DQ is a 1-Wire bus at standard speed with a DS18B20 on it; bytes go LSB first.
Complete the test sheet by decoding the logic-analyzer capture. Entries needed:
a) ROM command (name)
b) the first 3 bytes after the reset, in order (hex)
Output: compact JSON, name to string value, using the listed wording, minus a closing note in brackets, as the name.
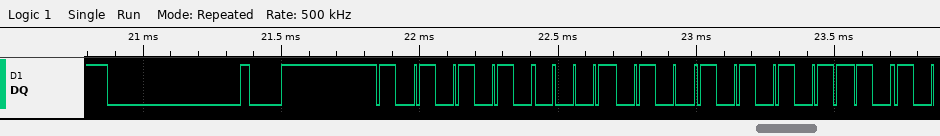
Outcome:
{"ROM command": "Match ROM", "the first 3 bytes after the reset, in order": "55 28 D5"}
